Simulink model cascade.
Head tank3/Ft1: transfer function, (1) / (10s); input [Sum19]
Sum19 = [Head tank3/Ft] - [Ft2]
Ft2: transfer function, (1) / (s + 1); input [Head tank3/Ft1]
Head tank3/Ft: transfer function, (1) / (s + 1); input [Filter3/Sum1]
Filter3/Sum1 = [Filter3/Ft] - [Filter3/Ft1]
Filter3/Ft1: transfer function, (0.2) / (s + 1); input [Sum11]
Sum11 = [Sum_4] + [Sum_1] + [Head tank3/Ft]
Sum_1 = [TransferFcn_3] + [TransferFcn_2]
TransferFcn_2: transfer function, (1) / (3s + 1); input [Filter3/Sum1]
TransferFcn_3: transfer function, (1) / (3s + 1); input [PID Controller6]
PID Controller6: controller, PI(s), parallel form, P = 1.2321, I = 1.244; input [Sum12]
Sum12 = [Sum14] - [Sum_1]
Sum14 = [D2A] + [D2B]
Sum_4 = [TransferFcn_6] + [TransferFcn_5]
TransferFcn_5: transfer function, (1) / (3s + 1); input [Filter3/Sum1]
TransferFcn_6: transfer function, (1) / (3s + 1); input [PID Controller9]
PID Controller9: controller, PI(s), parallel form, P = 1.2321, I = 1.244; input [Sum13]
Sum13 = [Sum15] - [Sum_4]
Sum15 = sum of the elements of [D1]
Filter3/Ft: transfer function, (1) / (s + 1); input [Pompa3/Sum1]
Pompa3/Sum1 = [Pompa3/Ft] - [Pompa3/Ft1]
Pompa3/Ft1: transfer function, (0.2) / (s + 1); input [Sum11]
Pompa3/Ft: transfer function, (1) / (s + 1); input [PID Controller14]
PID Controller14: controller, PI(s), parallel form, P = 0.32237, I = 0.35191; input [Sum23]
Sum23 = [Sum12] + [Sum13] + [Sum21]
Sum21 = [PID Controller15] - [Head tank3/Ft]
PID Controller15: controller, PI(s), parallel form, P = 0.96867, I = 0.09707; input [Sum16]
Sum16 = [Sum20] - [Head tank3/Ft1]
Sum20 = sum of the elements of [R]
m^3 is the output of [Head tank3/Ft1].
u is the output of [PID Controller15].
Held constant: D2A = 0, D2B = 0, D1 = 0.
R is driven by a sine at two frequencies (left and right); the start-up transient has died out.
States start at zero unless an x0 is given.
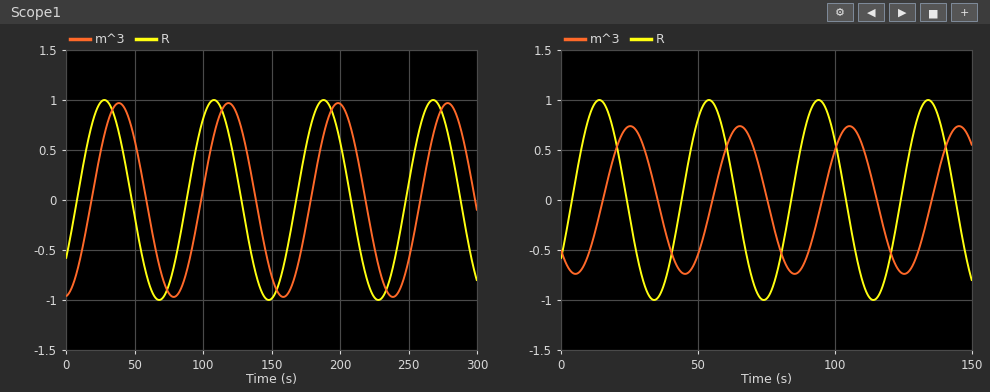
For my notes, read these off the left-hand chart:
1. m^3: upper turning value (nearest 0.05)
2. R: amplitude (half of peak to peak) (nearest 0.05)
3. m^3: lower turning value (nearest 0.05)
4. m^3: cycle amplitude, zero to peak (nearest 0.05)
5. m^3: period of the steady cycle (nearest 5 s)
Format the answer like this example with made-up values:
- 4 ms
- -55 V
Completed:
- 0.95
- 1.00
- -0.95
- 0.95
- 80 s
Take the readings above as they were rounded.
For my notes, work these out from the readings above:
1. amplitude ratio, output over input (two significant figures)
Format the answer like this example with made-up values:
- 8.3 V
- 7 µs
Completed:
- 0.95
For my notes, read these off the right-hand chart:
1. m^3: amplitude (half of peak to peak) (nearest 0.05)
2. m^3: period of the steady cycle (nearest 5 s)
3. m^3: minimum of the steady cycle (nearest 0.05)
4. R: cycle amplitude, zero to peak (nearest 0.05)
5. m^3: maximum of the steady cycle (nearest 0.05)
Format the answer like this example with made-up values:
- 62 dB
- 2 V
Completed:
- 0.75
- 40 s
- -0.75
- 1.00
- 0.75
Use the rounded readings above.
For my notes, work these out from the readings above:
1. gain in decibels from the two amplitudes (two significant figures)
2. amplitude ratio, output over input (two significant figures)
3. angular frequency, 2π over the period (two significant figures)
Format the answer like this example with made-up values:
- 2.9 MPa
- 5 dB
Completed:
- -2.5 dB
- 0.75
- 0.16 rad/s
